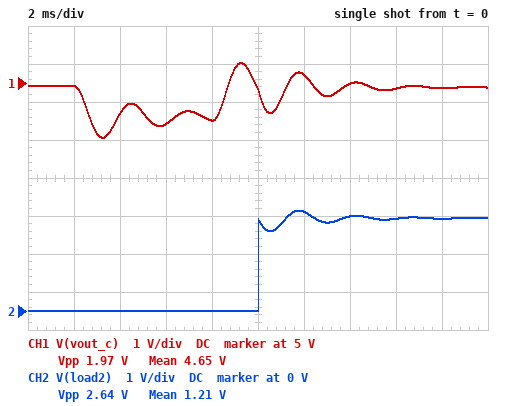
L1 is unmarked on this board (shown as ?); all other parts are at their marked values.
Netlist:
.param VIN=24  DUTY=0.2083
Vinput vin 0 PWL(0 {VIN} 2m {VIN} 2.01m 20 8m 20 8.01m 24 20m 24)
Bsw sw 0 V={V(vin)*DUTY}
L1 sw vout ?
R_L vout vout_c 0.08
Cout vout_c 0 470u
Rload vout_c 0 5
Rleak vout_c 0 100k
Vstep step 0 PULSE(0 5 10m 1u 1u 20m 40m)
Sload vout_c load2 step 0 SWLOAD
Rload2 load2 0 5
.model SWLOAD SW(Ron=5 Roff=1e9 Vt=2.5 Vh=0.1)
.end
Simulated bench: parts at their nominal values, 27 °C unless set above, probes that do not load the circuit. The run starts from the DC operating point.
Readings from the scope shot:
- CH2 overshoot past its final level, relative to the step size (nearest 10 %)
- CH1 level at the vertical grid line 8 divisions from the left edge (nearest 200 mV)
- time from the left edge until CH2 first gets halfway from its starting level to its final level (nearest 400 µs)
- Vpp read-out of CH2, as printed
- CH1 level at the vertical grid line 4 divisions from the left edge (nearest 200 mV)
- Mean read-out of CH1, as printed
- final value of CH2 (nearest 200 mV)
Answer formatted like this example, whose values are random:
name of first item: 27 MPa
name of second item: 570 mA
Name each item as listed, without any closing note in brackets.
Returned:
CH2 overshoot past its final level, relative to the step size: 10 %
CH1 level at the vertical grid line 8 divisions from the left edge: 4.8 V
time from the left edge until CH2 first gets halfway from its starting level to its final level: 10.0 ms
Vpp read-out of CH2, as printed: 2.64 V
CH1 level at the vertical grid line 4 divisions from the left edge: 4.0 V
Mean read-out of CH1, as printed: 4.65 V
final value of CH2: 2.4 V
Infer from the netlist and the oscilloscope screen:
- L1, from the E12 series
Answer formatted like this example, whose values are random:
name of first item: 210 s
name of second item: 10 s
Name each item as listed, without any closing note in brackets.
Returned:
L1, from the E12 series: 330 µH
